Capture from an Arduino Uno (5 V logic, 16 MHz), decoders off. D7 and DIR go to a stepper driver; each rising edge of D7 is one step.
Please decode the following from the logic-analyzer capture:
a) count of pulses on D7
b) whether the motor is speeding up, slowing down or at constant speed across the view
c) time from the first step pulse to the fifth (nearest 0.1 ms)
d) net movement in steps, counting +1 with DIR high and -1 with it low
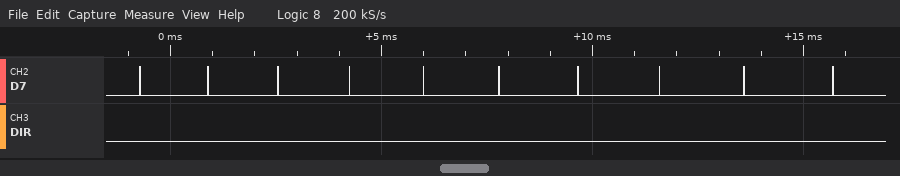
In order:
10
slowing down
6.7 ms
-10
